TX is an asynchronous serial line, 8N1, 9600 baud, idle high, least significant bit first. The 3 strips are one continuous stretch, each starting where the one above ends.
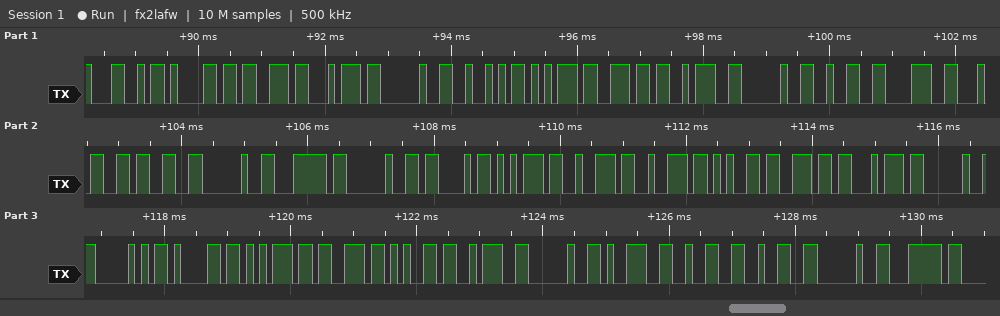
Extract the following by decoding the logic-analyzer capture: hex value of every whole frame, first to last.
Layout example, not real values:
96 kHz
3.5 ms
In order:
4C 61 73 74 20 52 75 6E 3A 20 32 38 34 33 20 7C 20 43 75 72 72 65 6E 74 20 50 61 75 73 65 3A 20 39 32 32 20 7C
